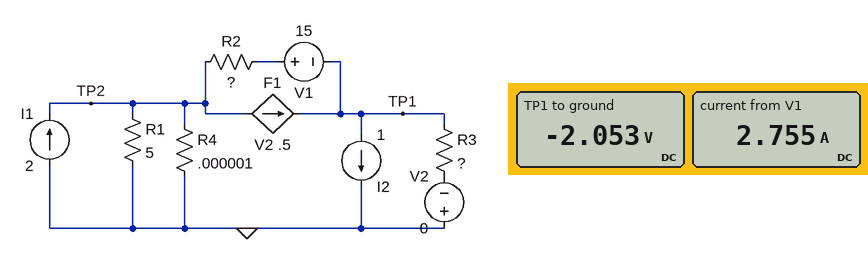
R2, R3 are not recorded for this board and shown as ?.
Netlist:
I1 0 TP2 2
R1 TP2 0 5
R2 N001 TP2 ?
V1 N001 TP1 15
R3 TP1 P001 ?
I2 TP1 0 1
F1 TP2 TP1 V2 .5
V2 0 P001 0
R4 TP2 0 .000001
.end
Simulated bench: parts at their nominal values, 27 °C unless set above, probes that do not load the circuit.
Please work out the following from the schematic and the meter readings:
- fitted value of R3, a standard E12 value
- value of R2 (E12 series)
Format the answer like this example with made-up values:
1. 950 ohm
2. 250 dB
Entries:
1. 0.82 Ω
2. 4.7 Ω
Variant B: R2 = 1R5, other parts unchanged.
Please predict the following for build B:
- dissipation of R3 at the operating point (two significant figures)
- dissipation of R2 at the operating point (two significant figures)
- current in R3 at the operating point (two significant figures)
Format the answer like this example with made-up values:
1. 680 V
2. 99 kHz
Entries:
1. 24 W
2. 75 W
3. 5.4 A
